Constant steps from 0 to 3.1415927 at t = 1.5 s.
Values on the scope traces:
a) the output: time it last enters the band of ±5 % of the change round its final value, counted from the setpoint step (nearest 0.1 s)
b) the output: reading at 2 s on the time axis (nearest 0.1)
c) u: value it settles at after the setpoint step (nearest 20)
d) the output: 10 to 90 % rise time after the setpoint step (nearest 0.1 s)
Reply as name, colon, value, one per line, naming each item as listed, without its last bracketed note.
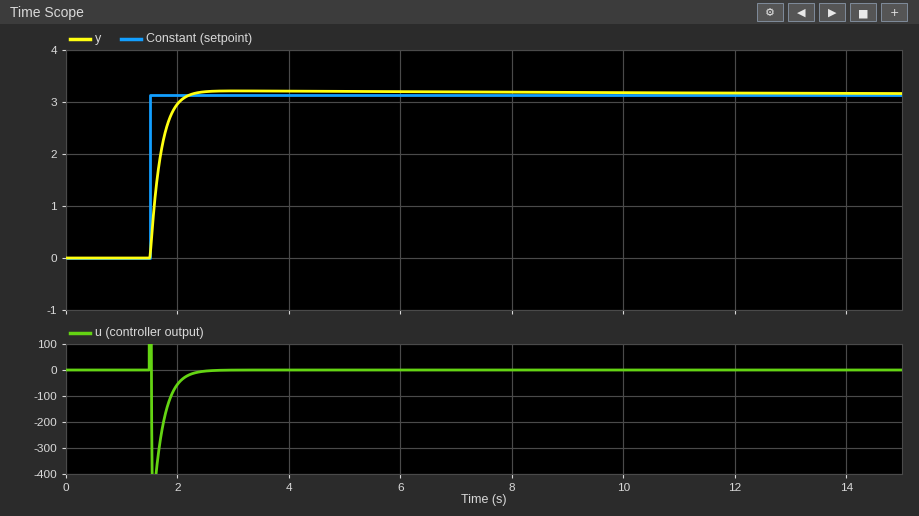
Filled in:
the output: time it last enters the band of ±5 % of the change round its final value, counted from the setpoint step: 0.5 s
the output: reading at 2 s on the time axis: 3.0
u: value it settles at after the setpoint step: 0
the output: 10 to 90 % rise time after the setpoint step: 0.4 s
